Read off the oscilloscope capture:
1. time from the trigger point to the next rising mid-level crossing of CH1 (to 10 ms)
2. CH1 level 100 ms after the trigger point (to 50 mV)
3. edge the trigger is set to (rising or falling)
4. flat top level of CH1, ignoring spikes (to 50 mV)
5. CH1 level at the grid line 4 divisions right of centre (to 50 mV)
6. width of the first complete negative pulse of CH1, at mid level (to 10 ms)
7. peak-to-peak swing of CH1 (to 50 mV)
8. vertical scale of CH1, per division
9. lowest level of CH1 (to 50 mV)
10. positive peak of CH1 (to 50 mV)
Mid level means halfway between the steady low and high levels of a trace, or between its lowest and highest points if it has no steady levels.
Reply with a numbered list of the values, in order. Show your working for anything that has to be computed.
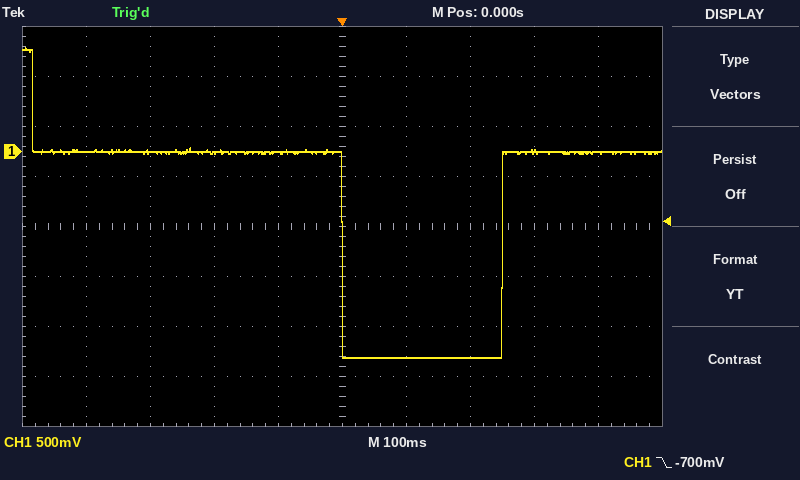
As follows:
1. 250 ms
2. -2.05 V
3. falling
4. 0 mV
5. 0 mV
6. 250 ms
7. 1.05 V − (-2.05 V) = 3.10 V
8. 500 mV
9. -2.05 V
10. 1.05 V
